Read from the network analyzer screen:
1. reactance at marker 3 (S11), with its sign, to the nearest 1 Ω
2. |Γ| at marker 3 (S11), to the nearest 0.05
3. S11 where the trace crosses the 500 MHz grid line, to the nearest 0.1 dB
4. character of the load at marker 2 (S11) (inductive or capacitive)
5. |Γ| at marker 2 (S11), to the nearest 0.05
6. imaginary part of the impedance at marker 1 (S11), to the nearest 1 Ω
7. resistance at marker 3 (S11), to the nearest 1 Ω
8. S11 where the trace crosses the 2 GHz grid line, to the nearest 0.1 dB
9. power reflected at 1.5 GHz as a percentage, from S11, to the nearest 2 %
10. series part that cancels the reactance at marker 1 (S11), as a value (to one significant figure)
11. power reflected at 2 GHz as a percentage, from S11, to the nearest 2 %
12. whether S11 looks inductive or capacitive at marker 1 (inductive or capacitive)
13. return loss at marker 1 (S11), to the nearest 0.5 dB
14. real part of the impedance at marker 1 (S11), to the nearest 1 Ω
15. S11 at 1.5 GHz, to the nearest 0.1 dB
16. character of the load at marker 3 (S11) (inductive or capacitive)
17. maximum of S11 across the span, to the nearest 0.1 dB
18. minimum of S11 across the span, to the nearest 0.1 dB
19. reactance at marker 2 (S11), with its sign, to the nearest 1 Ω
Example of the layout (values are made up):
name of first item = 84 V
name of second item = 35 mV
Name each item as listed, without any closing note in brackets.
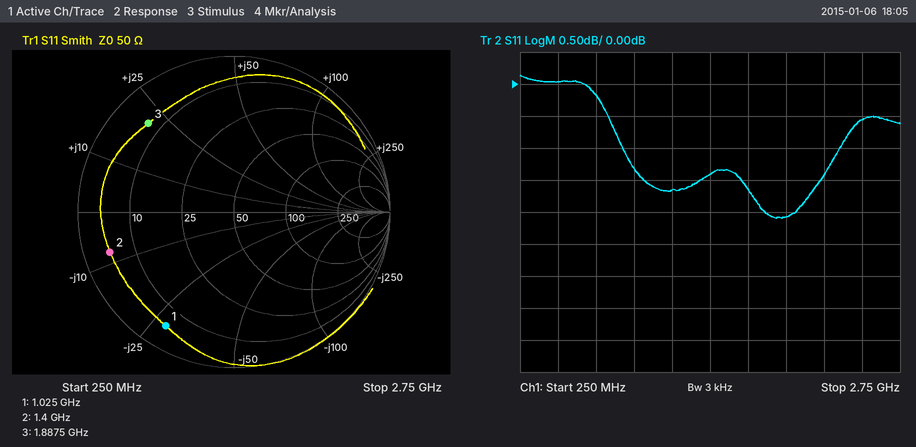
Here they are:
reactance at marker 3 (S11), with its sign, to the nearest 1 Ω = +21 Ω
|Γ| at marker 3 (S11), to the nearest 0.05 = 0.80
S11 where the trace crosses the 500 MHz grid line, to the nearest 0.1 dB = 0.0 dB
character of the load at marker 2 (S11) = capacitive
|Γ| at marker 2 (S11), to the nearest 0.05 = 0.85
imaginary part of the impedance at marker 1 (S11), to the nearest 1 Ω = -28 Ω
resistance at marker 3 (S11), to the nearest 1 Ω = 7 Ω
S11 where the trace crosses the 2 GHz grid line, to the nearest 0.1 dB = -2.1 dB
power reflected at 1.5 GHz as a percentage, from S11, to the nearest 2 % = 72 %
series part that cancels the reactance at marker 1 (S11), as a value = 4 nH
power reflected at 2 GHz as a percentage, from S11, to the nearest 2 % = 62 %
whether S11 looks inductive or capacitive at marker 1 = capacitive
return loss at marker 1 (S11), to the nearest 0.5 dB = 1.5 dB
real part of the impedance at marker 1 (S11), to the nearest 1 Ω = 5 Ω
S11 at 1.5 GHz, to the nearest 0.1 dB = -1.4 dB
character of the load at marker 3 (S11) = inductive
maximum of S11 across the span, to the nearest 0.1 dB = 0.1 dB
minimum of S11 across the span, to the nearest 0.1 dB = -2.1 dB
reactance at marker 2 (S11), with its sign, to the nearest 1 Ω = -8 Ω
